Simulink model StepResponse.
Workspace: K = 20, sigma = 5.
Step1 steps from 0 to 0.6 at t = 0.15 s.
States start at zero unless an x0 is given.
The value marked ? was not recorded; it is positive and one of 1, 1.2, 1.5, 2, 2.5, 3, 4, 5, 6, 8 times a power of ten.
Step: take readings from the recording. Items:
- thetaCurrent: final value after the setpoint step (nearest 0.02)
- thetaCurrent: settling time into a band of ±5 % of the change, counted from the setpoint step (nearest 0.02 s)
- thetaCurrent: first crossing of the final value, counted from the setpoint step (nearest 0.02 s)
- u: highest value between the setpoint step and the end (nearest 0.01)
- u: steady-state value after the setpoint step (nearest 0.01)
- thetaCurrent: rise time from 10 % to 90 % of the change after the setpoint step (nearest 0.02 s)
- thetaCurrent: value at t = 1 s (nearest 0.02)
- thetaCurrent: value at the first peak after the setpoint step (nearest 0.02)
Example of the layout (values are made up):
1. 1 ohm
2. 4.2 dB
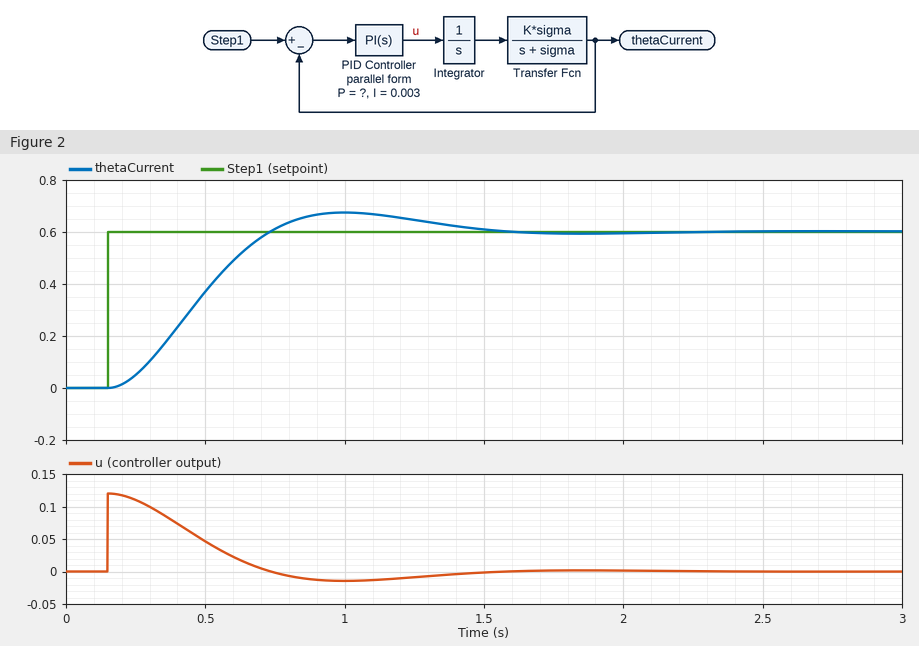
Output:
1. 0.60
2. 1.18 s
3. 0.58 s
4. 0.12
5. 0.00
6. 0.40 s
7. 0.68
8. 0.68
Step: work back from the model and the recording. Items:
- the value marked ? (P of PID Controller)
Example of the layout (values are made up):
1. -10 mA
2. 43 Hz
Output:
1. 0.2
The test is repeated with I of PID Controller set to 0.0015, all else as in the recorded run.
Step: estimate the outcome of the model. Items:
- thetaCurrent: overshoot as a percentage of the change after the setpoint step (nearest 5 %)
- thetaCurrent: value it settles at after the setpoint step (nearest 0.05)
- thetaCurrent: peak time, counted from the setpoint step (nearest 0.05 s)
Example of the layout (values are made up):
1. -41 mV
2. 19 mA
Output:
1. 10 %
2. 0.60
3. 0.85 s
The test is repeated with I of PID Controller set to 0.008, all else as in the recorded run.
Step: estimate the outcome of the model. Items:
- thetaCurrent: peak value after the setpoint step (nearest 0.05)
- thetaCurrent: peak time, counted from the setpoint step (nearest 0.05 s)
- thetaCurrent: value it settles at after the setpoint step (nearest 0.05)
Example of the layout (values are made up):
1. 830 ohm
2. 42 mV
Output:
1. 0.70
2. 0.85 s
3. 0.60
